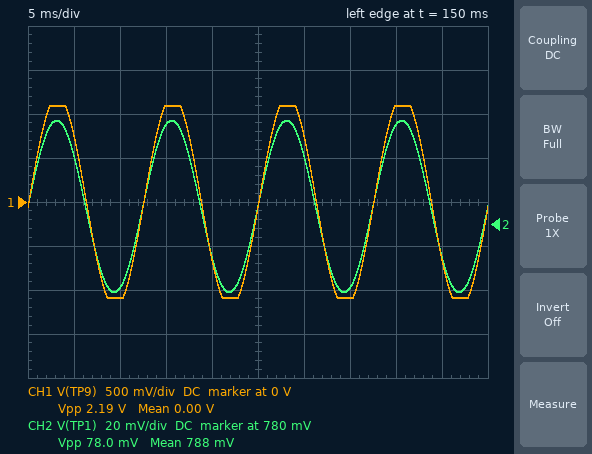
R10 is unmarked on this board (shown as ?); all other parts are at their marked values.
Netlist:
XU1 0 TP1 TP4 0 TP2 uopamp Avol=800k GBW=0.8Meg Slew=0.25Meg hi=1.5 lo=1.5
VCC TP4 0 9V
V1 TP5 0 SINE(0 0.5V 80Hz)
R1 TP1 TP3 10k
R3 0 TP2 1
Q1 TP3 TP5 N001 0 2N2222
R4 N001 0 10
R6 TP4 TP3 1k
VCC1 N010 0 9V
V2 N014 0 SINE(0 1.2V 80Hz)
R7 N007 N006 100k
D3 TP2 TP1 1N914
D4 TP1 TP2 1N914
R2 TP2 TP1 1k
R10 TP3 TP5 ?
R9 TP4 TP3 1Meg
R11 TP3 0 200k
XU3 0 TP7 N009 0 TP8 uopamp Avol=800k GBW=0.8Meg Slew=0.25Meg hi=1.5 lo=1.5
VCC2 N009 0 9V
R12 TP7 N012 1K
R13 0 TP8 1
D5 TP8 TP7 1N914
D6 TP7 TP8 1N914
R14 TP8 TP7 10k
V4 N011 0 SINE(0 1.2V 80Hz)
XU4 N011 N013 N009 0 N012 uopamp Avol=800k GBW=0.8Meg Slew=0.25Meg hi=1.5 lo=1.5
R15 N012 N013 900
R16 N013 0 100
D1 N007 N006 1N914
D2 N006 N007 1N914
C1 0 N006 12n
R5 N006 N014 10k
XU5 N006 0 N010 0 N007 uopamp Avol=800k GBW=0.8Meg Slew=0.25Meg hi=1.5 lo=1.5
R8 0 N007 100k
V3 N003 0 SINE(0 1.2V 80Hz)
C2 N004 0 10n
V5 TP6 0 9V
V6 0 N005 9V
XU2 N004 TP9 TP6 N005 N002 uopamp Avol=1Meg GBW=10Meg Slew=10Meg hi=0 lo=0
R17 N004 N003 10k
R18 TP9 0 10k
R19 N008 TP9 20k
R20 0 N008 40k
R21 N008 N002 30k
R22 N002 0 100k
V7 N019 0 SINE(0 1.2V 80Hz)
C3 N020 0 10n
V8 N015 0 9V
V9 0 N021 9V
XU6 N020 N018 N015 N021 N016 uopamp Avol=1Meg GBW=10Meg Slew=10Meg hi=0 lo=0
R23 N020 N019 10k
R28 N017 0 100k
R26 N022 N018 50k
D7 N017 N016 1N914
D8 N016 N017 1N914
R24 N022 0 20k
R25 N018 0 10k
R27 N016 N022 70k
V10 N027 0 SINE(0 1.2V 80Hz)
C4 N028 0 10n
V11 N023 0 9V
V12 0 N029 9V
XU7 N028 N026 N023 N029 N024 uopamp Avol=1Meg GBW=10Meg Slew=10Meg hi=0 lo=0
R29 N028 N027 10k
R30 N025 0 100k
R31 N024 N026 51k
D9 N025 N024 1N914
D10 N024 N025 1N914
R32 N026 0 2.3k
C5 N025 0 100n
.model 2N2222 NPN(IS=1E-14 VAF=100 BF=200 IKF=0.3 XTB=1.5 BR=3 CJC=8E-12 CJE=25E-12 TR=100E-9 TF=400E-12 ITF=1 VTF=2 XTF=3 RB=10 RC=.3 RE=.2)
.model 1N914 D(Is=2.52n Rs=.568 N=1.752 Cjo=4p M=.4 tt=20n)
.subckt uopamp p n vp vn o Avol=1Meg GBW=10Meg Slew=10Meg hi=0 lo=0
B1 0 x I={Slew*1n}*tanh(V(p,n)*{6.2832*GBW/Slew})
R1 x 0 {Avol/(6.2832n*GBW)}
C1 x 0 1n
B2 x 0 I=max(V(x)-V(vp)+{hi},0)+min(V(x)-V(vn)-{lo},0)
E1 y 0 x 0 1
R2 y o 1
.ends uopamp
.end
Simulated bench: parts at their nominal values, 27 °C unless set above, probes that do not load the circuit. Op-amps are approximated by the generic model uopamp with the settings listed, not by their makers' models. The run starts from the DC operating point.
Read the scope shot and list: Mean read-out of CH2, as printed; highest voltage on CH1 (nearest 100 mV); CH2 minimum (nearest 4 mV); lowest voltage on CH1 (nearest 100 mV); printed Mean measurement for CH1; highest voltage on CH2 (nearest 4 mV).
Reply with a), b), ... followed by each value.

a) 788 mV
b) 1.1 V
c) 748 mV
d) -1.1 V
e) 0.00 V
f) 828 mV
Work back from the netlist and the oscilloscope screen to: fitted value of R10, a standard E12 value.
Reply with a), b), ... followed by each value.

a) 150 Ω
